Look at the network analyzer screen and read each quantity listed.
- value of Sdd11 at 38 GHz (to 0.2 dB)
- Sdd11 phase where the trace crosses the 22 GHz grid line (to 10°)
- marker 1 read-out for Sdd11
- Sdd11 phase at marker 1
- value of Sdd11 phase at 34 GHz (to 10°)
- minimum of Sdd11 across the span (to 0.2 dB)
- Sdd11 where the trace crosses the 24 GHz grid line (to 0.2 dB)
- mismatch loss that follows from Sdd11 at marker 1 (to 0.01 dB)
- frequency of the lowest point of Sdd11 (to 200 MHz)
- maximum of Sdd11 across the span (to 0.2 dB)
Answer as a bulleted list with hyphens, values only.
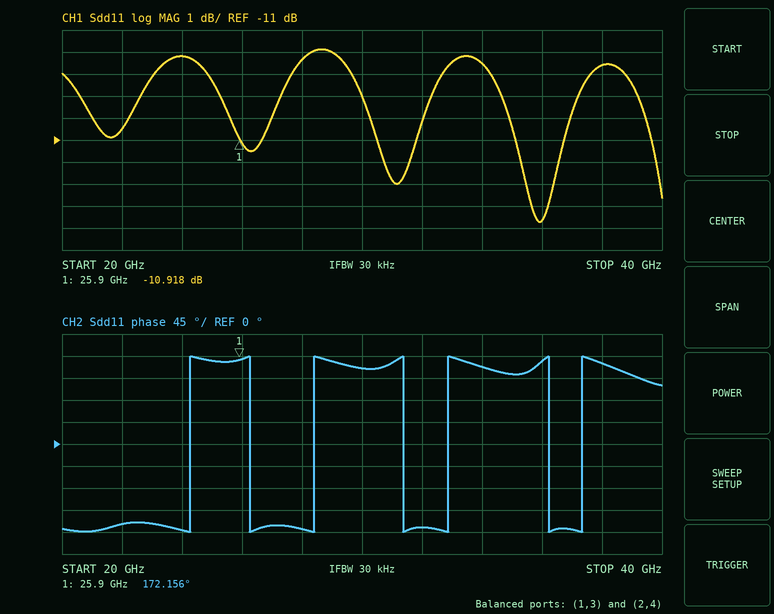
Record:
- -7.6 dB
- -160°
- -10.918 dB
- 172.156°
- 160°
- -14.8 dB
- -7.2 dB
- 0.37 dB
- 36.0 GHz
- -6.8 dB
